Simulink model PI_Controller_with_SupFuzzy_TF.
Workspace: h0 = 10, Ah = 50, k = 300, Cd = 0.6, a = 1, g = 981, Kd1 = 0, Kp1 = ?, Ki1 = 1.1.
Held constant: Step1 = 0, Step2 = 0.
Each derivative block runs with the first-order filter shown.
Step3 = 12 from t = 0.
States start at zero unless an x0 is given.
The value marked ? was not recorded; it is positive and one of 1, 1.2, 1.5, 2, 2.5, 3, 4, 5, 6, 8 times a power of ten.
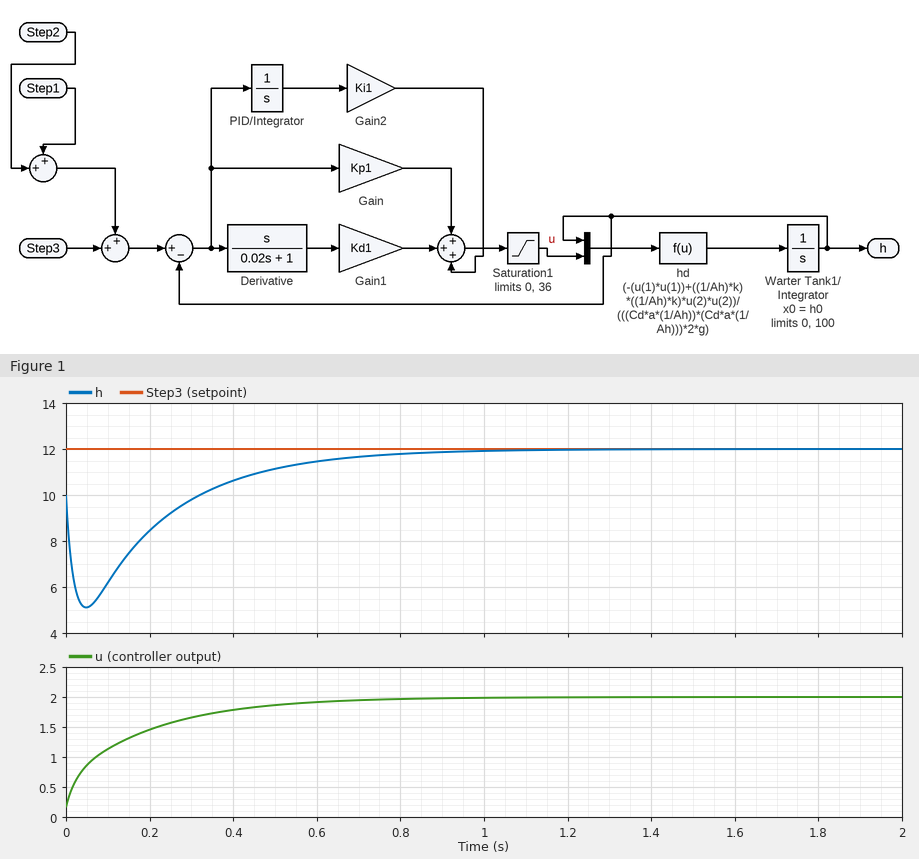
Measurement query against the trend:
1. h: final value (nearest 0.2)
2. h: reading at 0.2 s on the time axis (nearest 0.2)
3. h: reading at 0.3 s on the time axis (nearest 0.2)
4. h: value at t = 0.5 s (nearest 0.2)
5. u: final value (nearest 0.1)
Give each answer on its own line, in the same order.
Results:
12.0
8.4
9.8
11.2
2.0
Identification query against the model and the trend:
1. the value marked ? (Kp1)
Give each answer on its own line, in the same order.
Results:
0.08
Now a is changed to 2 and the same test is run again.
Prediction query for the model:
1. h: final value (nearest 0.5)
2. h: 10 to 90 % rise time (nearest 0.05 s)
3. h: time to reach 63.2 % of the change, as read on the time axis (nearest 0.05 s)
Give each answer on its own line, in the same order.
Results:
12.0
0.40 s
0.50 s
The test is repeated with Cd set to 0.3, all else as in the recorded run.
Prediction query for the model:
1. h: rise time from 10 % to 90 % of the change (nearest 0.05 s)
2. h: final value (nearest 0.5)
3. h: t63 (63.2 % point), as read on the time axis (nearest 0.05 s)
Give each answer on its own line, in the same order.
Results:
0.50 s
12.0
0.55 s
